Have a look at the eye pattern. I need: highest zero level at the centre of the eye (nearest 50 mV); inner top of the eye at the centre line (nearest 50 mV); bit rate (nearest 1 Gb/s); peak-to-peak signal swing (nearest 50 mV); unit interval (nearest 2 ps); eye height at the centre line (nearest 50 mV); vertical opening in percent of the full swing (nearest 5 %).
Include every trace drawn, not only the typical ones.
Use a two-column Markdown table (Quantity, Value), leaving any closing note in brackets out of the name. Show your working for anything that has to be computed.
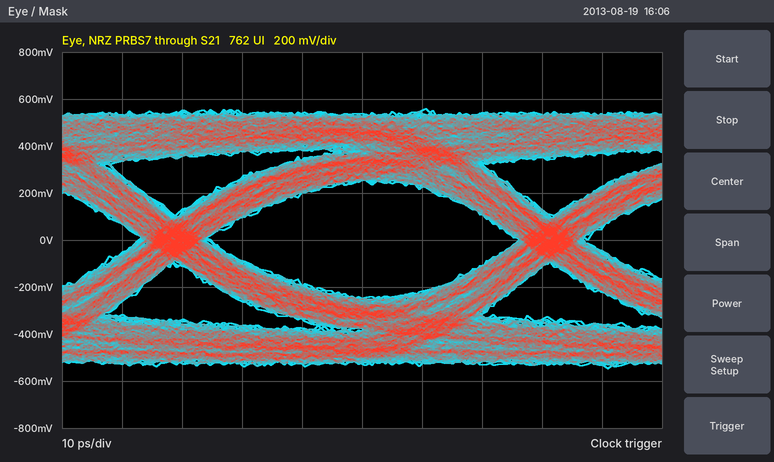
| Quantity | Value |
|---|---|
| highest zero level at the centre of the eye | -250 mV |
| inner top of the eye at the centre line | 250 mV |
| bit rate | 16 Gb/s |
| peak-to-peak signal swing | 1.10 V |
| unit interval | 62 ps |
| eye height at the centre line | 500 mV |
| vertical opening in percent of the full swing | 500 mV / 1.10 V ≈ 45 % |
